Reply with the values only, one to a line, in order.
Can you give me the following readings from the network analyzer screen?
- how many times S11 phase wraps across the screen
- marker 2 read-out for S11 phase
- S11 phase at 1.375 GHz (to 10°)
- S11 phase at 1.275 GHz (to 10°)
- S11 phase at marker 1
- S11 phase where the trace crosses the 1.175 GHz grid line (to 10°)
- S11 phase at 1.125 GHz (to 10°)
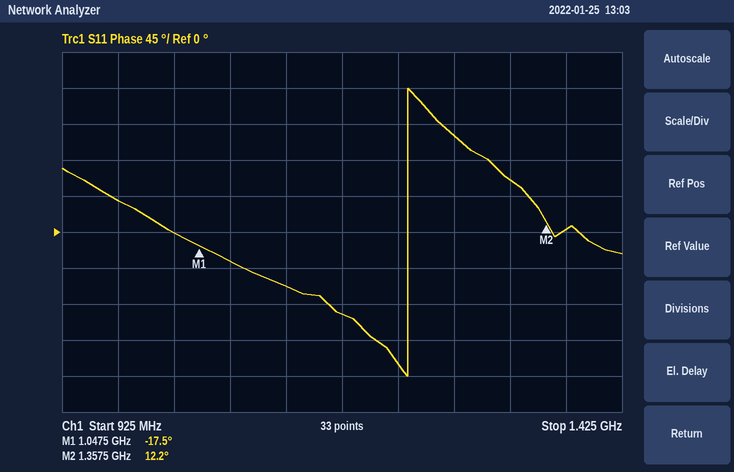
1
12.2°
0°
120°
-17.5°
-100°
-70°
